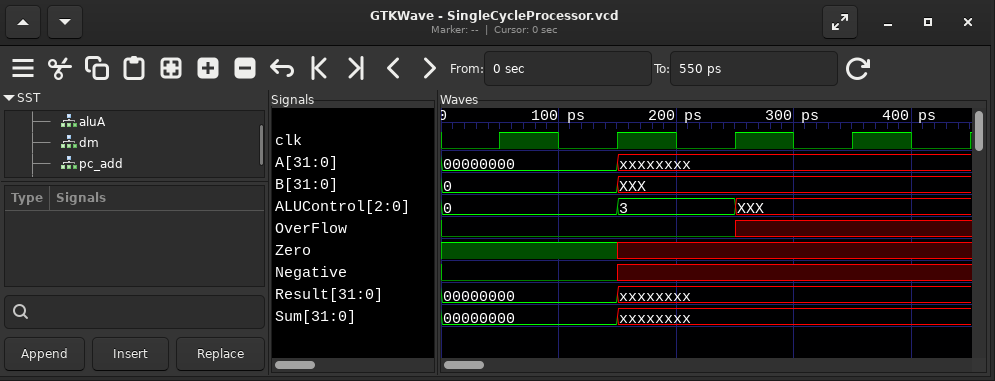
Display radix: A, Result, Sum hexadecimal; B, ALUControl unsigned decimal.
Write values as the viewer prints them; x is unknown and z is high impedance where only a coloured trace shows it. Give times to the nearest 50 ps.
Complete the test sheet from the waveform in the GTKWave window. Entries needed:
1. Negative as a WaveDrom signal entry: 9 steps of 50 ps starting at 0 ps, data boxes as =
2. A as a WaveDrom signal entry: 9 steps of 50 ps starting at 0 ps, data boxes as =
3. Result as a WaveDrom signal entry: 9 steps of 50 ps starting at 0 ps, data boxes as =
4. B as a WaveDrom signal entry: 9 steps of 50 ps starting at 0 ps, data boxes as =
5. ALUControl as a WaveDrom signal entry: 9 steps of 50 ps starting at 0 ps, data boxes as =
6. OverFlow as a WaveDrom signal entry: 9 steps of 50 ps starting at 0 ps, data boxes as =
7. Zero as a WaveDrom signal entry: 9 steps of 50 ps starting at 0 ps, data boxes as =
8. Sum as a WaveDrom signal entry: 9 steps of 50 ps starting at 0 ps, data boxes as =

{name: 'Negative', wave: '0..x.....'}
{name: 'A', wave: '=..x.....', data: '00000000'}
{name: 'Result', wave: '=..x.....', data: '00000000'}
{name: 'B', wave: '=..x.....', data: '0'}
{name: 'ALUControl', wave: '=..=.x...', data: '0 3'}
{name: 'OverFlow', wave: '0....x...'}
{name: 'Zero', wave: '1..x.....'}
{name: 'Sum', wave: '=..x.....', data: '00000000'}
